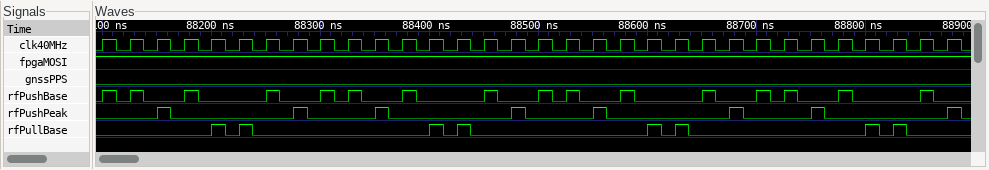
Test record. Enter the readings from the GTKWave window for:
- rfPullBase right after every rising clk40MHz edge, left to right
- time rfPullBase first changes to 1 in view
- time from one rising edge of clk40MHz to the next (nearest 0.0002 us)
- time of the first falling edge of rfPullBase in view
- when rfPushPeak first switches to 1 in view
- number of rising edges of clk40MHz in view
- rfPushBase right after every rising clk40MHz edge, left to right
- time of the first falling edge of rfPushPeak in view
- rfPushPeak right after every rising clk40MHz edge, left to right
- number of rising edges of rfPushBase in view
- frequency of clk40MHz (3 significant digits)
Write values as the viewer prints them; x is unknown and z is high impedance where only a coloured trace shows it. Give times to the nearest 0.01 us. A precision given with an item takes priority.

0 0 0 0 1 1 0 0 0 0 0 0 1 1 0 0 0 0 0 0 1 1 0 0 0 0 0 0 1 1 0 0
88.2 us
0.025 us
88.21 us
88.15 us
32
1 1 0 1 0 0 1 0 1 1 0 1 0 0 1 0 1 1 0 1 0 0 1 0 1 1 0 1 0 0 1 0
88.16 us
0 0 1 0 0 0 0 1 0 0 1 0 0 0 0 1 0 0 1 0 0 0 0 1 0 0 1 0 0 0 0 1
16
40.0 MHz
